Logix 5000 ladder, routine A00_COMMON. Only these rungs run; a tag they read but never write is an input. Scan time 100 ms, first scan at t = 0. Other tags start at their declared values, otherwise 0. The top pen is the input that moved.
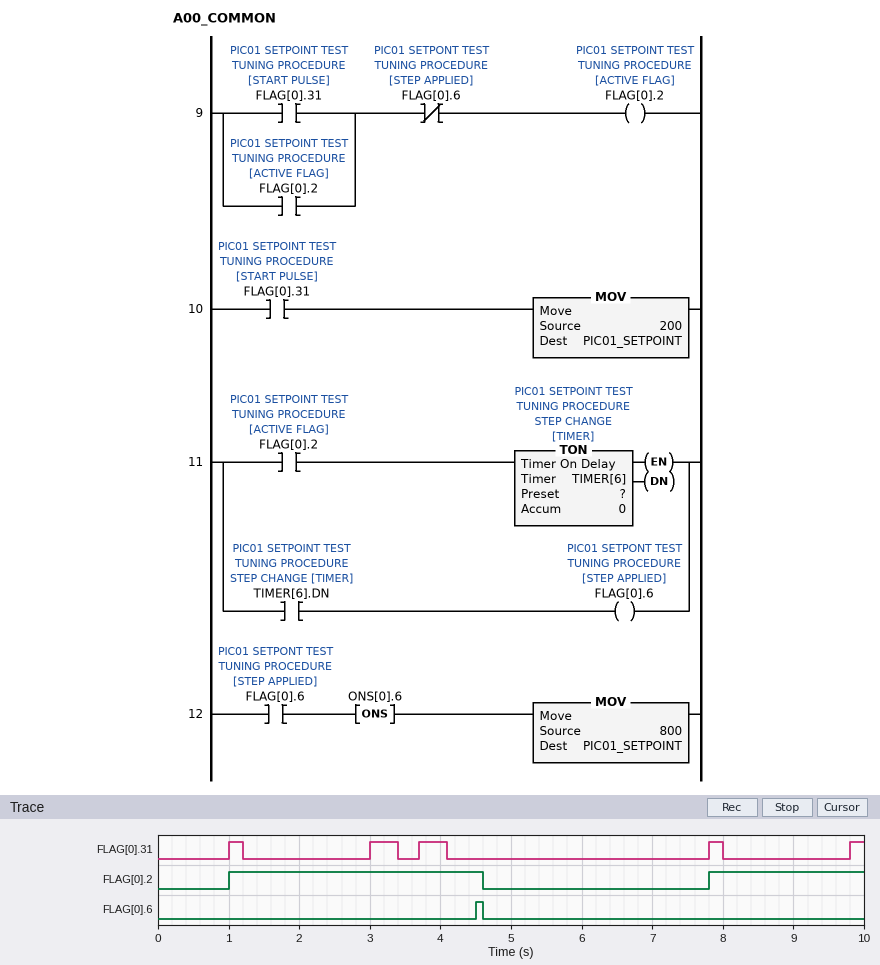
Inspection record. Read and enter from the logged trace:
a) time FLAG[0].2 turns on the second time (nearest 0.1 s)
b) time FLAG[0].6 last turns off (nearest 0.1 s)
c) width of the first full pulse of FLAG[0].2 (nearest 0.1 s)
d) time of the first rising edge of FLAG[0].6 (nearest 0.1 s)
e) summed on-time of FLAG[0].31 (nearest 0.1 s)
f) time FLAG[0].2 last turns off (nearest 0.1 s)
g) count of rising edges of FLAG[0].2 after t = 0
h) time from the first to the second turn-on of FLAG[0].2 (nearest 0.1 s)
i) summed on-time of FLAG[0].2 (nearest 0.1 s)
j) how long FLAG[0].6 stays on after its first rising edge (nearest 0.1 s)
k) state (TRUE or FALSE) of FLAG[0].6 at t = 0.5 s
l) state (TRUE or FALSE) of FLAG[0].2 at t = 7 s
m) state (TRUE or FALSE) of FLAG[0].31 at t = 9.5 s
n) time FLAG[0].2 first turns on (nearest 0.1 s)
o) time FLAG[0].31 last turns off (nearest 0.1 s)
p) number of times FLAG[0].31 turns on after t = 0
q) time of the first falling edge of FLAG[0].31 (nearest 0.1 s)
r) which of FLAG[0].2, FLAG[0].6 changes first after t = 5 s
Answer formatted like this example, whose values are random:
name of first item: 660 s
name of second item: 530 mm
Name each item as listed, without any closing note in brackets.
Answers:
time FLAG[0].2 turns on the second time: 7.8 s
time FLAG[0].6 last turns off: 4.6 s
width of the first full pulse of FLAG[0].2: 3.6 s
time of the first rising edge of FLAG[0].6: 4.5 s
summed on-time of FLAG[0].31: 1.4 s
time FLAG[0].2 last turns off: 4.6 s
count of rising edges of FLAG[0].2 after t = 0: 2
time from the first to the second turn-on of FLAG[0].2: 6.8 s
summed on-time of FLAG[0].2: 5.8 s
how long FLAG[0].6 stays on after its first rising edge: 0.1 s
state (TRUE or FALSE) of FLAG[0].6 at t = 0.5 s: FALSE
state (TRUE or FALSE) of FLAG[0].2 at t = 7 s: FALSE
state (TRUE or FALSE) of FLAG[0].31 at t = 9.5 s: FALSE
time FLAG[0].2 first turns on: 1.0 s
time FLAG[0].31 last turns off: 8.0 s
number of times FLAG[0].31 turns on after t = 0: 5
time of the first falling edge of FLAG[0].31: 1.2 s
which of FLAG[0].2, FLAG[0].6 changes first after t = 5 s: FLAG[0].2
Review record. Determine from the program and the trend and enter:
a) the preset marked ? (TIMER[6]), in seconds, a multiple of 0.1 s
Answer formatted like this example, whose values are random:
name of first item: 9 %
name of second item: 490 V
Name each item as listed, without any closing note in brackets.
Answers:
the preset marked ? (TIMER[6]), in seconds, a multiple of 0.1 s: 3.5 s
